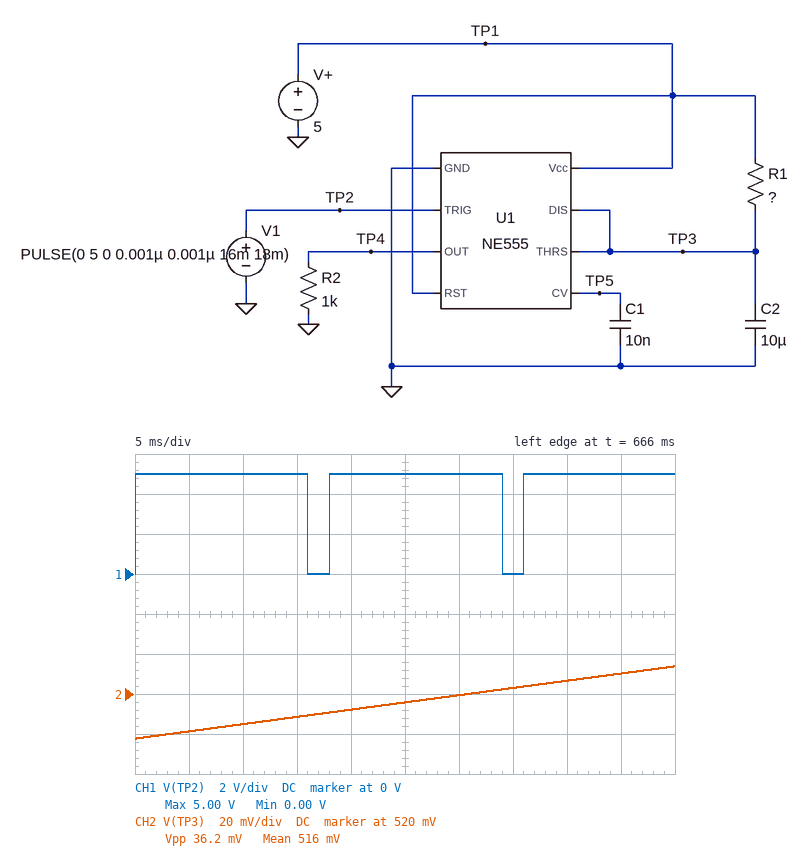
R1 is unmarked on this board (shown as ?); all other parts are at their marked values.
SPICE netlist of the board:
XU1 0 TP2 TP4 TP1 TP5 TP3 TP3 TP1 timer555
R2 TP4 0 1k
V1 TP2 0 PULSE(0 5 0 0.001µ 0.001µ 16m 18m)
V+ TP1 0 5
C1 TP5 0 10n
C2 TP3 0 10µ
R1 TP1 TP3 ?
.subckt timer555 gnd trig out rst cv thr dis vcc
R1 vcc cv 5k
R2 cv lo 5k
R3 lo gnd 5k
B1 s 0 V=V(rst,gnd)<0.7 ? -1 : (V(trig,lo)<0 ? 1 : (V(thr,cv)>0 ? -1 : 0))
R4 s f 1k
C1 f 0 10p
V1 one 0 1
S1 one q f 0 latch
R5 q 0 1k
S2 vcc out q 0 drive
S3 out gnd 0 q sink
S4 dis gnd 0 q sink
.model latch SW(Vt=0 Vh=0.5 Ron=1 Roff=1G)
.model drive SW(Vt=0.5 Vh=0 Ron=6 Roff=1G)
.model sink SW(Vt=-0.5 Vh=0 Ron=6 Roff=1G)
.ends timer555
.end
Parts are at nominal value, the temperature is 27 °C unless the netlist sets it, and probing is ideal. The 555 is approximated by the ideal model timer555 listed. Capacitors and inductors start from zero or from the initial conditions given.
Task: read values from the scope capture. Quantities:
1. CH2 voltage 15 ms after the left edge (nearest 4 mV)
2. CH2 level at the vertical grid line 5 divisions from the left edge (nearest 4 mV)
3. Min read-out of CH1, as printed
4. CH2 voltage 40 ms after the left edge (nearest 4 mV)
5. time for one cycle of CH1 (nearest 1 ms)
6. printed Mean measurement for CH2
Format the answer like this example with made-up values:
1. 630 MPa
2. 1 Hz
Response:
1. 508 mV
2. 516 mV
3. 0.00 V
4. 528 mV
5. 18 ms
6. 516 mV
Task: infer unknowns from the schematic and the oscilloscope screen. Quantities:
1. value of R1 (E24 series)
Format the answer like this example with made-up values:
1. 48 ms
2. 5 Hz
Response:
1. 620 kΩ
